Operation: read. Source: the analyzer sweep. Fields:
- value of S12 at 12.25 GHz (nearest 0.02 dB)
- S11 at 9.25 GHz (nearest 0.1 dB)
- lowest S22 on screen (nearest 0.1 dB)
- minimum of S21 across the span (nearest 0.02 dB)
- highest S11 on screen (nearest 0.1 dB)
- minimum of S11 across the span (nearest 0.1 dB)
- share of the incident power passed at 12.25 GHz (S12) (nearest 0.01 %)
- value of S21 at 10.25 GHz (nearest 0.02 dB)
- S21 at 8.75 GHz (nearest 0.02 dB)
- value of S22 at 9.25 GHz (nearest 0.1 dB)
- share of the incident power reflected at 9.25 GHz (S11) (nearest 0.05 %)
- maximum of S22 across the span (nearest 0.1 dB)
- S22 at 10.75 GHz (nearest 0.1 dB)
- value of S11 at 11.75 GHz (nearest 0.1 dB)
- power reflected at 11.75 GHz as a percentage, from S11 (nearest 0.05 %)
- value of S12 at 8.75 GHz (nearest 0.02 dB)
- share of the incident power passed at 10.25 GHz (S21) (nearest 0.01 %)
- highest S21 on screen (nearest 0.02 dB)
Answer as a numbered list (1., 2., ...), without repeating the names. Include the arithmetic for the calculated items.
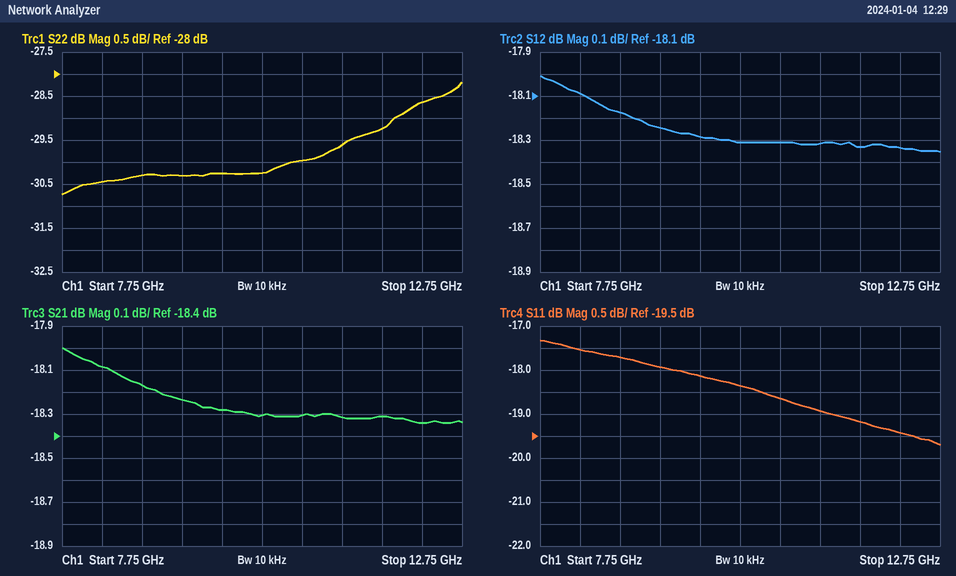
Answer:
1. -18.34 dB
2. -17.9 dB
3. -30.7 dB
4. -18.34 dB
5. -17.3 dB
6. -19.7 dB
7. 10^(-18.34/10) ≈ 1.47 %
8. -18.30 dB
9. -18.16 dB
10. -30.3 dB
11. 10^(-17.9/10) ≈ 1.62 %, so 1.60 % to the nearest 0.05 %
12. -28.2 dB
13. -30.0 dB
14. -19.2 dB
15. 10^(-19.2/10) ≈ 1.20 %
16. -18.18 dB
17. 10^(-18.3/10) ≈ 1.48 %
18. -18.00 dB
